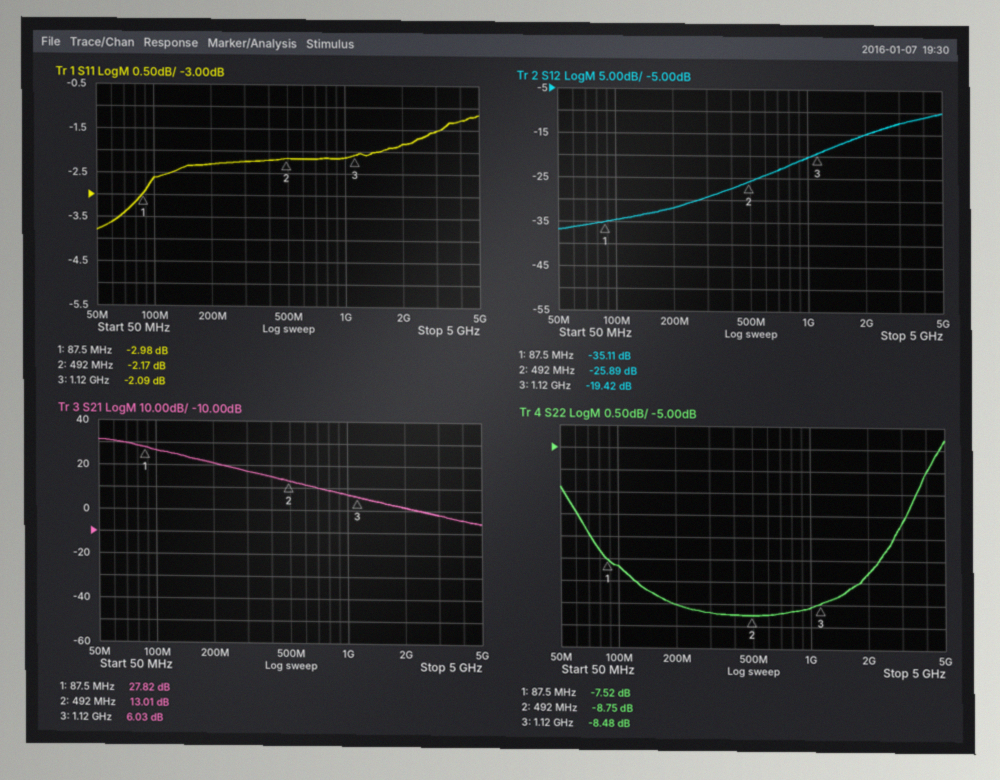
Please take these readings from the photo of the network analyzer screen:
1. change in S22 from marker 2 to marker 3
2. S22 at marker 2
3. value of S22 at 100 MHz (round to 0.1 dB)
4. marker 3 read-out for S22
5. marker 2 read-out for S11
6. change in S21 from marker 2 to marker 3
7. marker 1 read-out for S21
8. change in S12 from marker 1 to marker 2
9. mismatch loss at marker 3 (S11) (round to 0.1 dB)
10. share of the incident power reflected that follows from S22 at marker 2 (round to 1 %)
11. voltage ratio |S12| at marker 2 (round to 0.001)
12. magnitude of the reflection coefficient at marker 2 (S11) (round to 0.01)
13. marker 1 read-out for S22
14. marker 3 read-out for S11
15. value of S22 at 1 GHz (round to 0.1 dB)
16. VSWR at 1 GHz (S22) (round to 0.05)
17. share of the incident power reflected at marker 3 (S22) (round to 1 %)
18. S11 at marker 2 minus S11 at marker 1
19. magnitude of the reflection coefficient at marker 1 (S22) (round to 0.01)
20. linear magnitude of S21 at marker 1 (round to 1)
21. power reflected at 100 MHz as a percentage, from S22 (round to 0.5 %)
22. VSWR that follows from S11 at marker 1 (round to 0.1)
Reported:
0.27 dB
-8.75 dB
-7.7 dB
-8.48 dB
-2.17 dB
-6.98 dB
27.82 dB
9.22 dB
4.2 dB
13 %
0.051
0.78
-7.52 dB
-2.09 dB
-8.6 dB
2.20
14 %
0.81 dB
0.42
25
17.0 %
5.9
